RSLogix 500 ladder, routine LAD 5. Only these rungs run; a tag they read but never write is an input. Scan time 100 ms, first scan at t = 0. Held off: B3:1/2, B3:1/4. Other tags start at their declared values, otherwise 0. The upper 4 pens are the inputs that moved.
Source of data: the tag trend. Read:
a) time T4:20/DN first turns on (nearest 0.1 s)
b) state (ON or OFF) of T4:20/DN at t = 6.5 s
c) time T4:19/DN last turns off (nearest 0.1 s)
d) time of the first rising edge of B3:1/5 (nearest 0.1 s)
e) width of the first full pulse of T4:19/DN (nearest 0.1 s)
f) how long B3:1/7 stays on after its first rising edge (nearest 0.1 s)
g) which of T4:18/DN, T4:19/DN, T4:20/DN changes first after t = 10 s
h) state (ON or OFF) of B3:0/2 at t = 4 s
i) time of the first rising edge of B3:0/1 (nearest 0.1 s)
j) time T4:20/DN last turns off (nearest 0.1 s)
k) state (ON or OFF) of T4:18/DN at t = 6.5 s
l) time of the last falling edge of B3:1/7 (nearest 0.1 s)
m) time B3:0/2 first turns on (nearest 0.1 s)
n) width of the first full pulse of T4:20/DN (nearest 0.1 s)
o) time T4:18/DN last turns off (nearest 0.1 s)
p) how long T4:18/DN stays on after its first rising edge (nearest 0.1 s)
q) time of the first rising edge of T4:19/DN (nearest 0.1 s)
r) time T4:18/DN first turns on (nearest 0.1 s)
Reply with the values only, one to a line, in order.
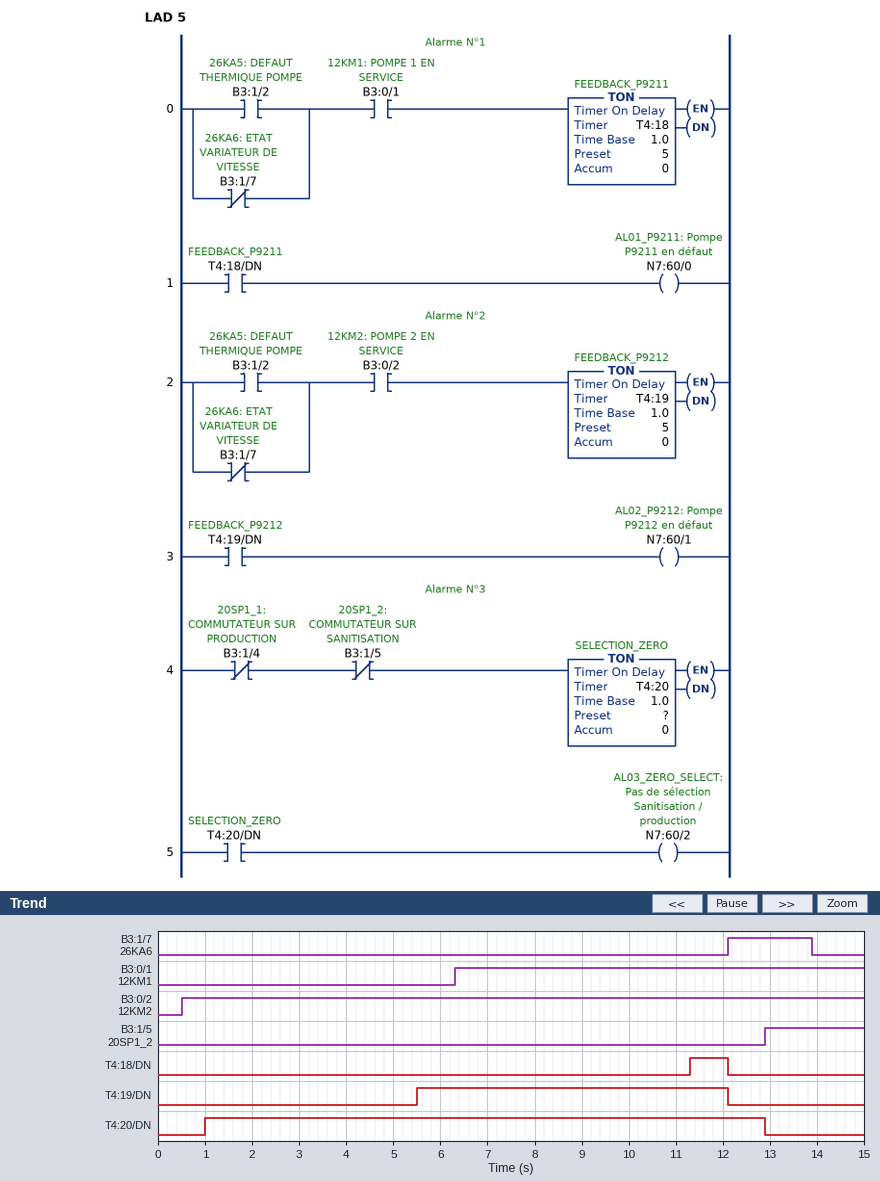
1.0 s
ON
12.1 s
12.9 s
6.6 s
1.8 s
T4:18/DN
ON
6.3 s
12.9 s
OFF
13.9 s
0.5 s
11.9 s
12.1 s
0.8 s
5.5 s
11.3 s
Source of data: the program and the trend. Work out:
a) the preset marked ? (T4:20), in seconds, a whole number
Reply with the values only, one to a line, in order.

1 s
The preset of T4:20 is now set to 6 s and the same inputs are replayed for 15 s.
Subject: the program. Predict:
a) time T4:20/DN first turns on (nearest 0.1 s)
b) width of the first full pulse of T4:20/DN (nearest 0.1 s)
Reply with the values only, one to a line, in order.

6.0 s
6.9 s
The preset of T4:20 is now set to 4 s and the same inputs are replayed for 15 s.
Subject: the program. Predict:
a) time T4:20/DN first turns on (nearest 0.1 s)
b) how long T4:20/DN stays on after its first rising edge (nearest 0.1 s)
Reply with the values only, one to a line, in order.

4.0 s
8.9 s
